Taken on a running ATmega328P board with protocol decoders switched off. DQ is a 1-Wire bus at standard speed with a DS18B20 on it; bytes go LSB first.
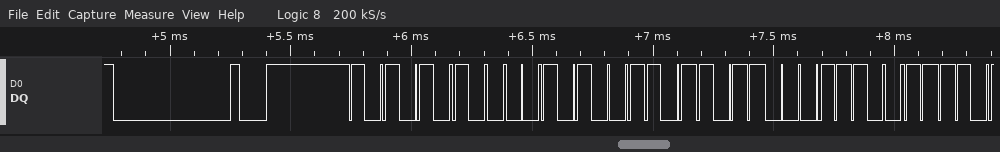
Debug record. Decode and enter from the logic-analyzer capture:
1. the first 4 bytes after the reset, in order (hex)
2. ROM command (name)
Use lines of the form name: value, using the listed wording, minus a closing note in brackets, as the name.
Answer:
the first 4 bytes after the reset, in order: 55 28 DB 38
ROM command: Match ROM
